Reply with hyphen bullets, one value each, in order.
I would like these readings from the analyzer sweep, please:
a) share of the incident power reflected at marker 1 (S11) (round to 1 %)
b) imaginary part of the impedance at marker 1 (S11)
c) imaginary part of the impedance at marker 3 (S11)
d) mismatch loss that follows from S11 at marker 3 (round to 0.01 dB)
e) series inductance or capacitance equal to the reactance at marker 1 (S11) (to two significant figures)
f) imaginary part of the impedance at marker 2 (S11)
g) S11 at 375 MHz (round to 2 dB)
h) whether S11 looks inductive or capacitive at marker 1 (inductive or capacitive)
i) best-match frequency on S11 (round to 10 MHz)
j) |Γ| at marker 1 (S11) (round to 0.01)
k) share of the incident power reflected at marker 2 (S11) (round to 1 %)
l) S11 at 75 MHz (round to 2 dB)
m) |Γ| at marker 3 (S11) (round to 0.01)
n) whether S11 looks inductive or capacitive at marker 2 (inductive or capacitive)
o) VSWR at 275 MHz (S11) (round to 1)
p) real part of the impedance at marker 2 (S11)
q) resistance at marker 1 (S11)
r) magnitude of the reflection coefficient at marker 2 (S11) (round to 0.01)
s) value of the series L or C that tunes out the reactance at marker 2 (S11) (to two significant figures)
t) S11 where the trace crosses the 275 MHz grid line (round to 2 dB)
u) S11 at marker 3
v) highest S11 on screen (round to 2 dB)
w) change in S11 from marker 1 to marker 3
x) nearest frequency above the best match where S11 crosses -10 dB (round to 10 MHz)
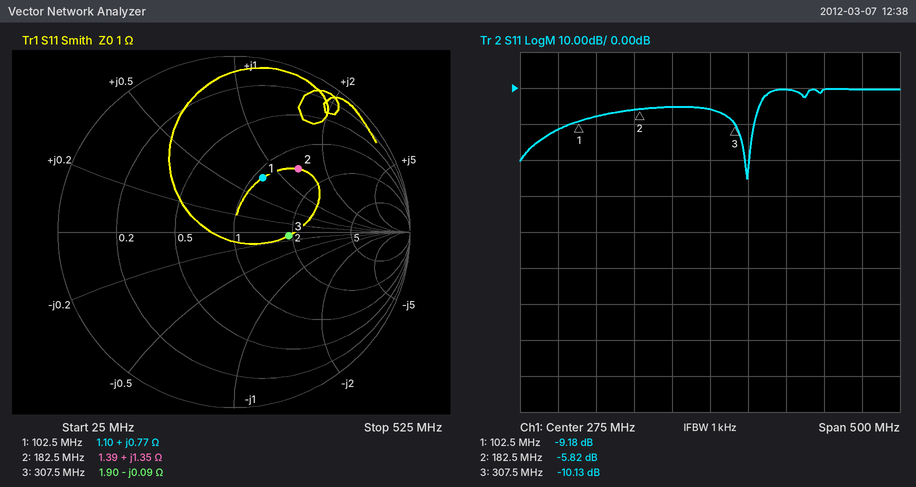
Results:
- 12 %
- +0.77 Ω
- -0.09 Ω
- 0.44 dB
- 1.2 nH
- +1.35 Ω
- 0 dB
- inductive
- 320 MHz
- 0.35
- 26 %
- -12 dB
- 0.31
- inductive
- 3
- 1.39 Ω
- 1.10 Ω
- 0.51
- 650 pF
- -6 dB
- -10.13 dB
- 0 dB
- -0.95 dB
- 330 MHz
